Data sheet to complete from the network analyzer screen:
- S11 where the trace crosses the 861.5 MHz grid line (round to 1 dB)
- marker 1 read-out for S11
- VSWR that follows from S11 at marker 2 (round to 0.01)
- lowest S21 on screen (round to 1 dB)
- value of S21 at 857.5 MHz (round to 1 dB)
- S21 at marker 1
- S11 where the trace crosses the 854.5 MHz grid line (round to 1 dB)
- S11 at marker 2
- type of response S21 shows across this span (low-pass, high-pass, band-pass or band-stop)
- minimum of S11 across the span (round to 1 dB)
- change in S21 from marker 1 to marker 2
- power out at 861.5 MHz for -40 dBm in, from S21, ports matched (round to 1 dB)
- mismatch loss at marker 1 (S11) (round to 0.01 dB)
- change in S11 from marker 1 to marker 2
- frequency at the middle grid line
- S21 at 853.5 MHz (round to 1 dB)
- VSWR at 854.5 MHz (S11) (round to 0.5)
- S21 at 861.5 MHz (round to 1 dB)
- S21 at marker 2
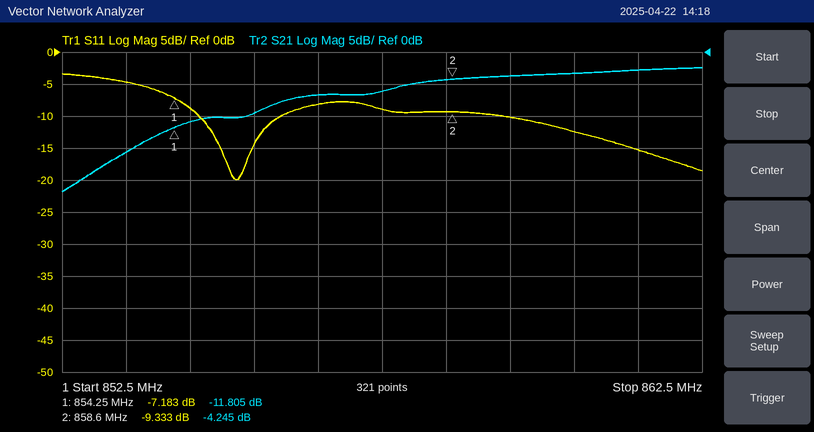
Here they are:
-15 dB
-7.183 dB
2.04
-22 dB
-6 dB
-11.805 dB
-9 dB
-9.333 dB
high-pass
-20 dB
7.560 dB
-43 dBm
0.92 dB
-2.150 dB
857.5 MHz
-16 dB
2.0
-3 dB
-4.245 dB
